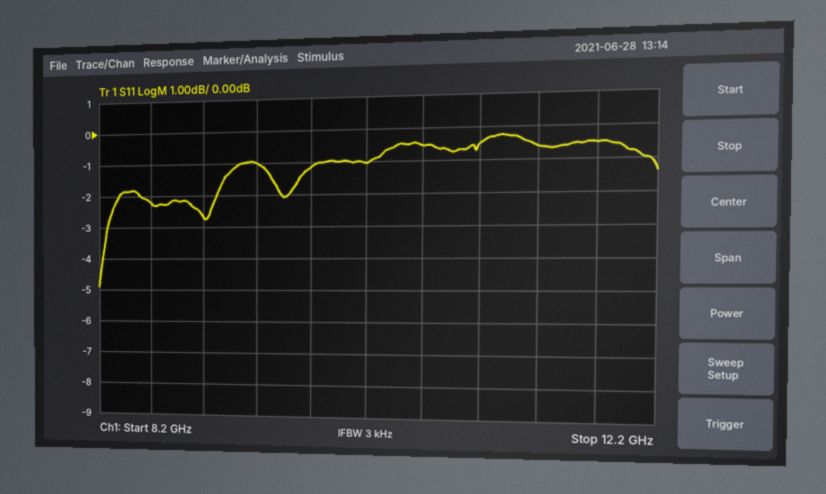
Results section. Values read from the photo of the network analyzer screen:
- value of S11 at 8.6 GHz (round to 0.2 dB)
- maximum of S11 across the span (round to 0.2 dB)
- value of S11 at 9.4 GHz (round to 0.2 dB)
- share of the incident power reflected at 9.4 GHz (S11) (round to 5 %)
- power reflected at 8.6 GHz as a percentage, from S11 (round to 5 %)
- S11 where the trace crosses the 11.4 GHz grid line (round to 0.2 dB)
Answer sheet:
-2.2 dB
-0.2 dB
-1.0 dB
80 %
60 %
-0.6 dB
